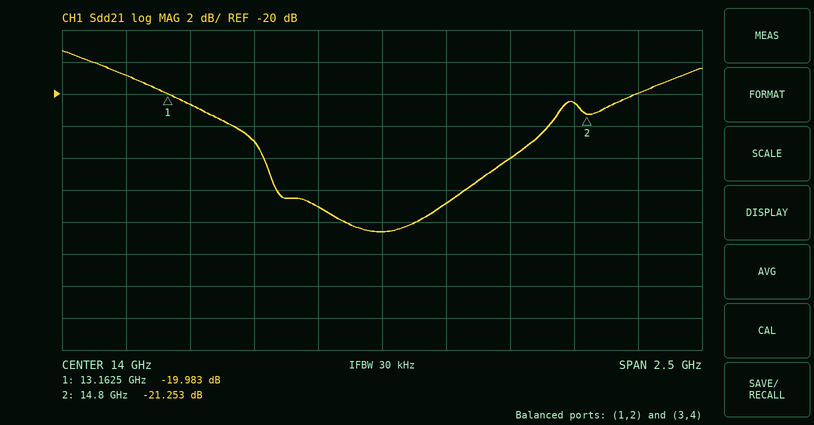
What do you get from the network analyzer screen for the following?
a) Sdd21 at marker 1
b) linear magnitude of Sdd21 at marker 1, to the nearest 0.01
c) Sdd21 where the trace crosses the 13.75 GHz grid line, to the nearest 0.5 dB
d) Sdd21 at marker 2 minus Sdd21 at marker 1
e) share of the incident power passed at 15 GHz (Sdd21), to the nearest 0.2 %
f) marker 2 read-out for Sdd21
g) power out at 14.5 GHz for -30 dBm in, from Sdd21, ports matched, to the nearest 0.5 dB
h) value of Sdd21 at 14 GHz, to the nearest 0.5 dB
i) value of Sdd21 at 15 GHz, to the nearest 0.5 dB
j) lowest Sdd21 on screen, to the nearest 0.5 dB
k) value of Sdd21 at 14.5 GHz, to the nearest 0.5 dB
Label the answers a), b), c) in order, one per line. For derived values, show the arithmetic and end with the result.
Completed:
a) -19.983 dB
b) 10^(-19.983/20) ≈ 0.10
c) -27.0 dB
d) -21.253 − (-19.983) = -1.270 dB
e) 10^(-20/10) ≈ 1.0 %
f) -21.253 dB
g) -30 dBm + (-24.0 dB) = -54.0 dBm
h) -28.5 dB
i) -20.0 dB
j) -28.5 dB
k) -24.0 dB
